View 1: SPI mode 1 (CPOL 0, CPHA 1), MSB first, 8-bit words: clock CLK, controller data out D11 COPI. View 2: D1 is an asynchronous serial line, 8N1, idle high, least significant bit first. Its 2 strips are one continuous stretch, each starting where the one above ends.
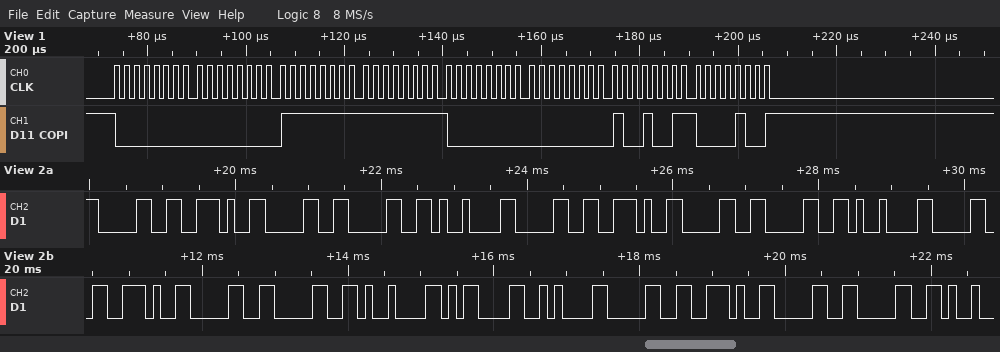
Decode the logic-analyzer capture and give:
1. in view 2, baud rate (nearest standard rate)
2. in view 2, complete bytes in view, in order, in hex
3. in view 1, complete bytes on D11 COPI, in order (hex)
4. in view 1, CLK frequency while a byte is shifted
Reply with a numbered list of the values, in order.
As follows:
1. 9600 baud
2. 0x30 0x2E 0x30 0x30 0x09 0x30 0x2E 0x30 0x30 0x09 0x30 0x2E 0x30 0x30 0x09 0x0D 0x0A 0x30 0x2E 0x30 0x30
3. 00 00 FF FF 00 00 93 09
4. 500 kHz
